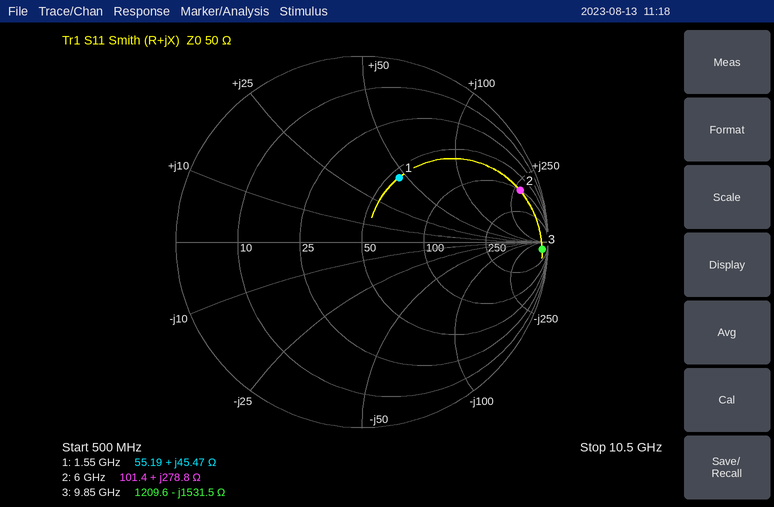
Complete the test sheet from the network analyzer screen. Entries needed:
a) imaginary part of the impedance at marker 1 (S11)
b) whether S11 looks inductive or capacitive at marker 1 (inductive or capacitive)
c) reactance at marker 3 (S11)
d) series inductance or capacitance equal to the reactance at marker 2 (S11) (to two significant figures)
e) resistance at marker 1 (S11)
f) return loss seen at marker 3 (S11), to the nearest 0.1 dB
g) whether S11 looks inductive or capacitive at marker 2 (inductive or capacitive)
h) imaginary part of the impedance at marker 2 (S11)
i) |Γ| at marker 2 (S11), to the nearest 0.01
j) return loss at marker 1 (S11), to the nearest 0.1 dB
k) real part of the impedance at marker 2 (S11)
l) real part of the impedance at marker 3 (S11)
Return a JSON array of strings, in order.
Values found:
["+45.47 Ω", "inductive", "-1531.5 Ω", "7.4 nH", "55.19 Ω", "0.3 dB", "inductive", "+278.8 Ω", "0.89", "8.0 dB", "101.4 Ω", "1209.6 Ω"]
